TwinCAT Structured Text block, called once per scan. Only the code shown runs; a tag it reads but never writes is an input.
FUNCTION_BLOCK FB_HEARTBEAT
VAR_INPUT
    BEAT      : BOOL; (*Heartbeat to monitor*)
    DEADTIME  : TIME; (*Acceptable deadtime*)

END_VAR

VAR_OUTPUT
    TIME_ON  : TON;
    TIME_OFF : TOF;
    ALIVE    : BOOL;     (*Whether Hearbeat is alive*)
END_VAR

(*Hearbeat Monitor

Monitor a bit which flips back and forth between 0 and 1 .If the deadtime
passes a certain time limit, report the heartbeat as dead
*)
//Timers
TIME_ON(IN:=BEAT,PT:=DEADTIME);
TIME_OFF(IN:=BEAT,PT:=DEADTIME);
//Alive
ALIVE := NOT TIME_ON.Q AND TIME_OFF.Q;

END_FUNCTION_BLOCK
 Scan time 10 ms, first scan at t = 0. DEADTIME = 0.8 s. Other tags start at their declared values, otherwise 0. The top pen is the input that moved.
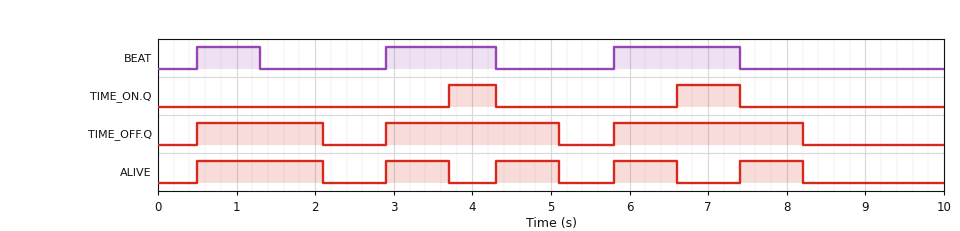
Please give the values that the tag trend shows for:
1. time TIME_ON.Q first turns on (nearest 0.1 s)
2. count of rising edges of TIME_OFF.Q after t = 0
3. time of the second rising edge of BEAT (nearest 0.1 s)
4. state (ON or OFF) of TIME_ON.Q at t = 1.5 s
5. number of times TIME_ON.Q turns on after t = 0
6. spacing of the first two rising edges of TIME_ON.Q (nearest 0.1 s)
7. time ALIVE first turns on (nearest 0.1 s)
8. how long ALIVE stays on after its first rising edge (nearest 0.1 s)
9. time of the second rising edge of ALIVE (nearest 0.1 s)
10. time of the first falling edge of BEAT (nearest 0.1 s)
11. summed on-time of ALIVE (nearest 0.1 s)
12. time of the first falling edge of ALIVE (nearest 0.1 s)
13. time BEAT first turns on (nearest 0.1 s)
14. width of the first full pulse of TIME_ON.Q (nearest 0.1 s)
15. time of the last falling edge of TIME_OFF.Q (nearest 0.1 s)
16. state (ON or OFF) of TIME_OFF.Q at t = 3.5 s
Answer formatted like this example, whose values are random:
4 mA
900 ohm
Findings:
3.7 s
3
2.9 s
OFF
2
2.9 s
0.5 s
1.6 s
2.9 s
1.3 s
4.8 s
2.1 s
0.5 s
0.6 s
8.2 s
ON
